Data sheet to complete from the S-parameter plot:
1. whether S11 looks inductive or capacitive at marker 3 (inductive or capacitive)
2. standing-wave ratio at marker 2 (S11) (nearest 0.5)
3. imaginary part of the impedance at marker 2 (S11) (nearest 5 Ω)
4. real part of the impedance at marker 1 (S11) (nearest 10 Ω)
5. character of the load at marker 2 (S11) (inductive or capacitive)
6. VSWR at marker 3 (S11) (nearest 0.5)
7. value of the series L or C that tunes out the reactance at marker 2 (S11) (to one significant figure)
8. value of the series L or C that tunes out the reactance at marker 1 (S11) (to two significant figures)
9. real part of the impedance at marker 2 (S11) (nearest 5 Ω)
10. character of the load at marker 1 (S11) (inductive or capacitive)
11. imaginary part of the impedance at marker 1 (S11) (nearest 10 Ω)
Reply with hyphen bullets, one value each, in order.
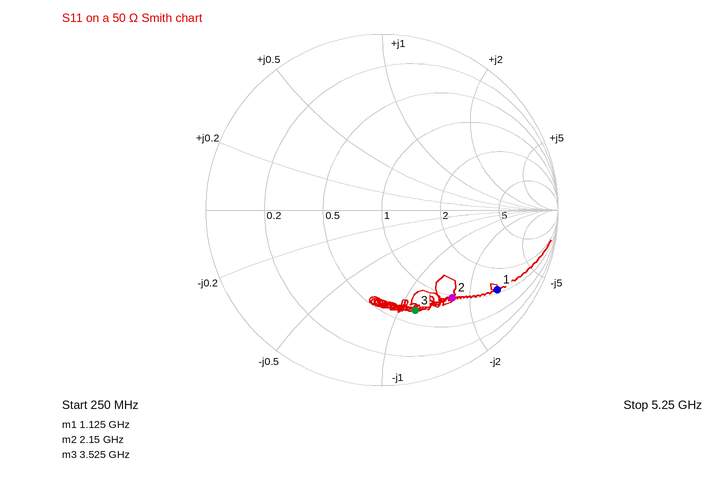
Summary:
- capacitive
- 4.5
- -80 Ω
- 60 Ω
- capacitive
- 4.0
- 6 nH
- 20 nH
- 50 Ω
- capacitive
- -140 Ω
